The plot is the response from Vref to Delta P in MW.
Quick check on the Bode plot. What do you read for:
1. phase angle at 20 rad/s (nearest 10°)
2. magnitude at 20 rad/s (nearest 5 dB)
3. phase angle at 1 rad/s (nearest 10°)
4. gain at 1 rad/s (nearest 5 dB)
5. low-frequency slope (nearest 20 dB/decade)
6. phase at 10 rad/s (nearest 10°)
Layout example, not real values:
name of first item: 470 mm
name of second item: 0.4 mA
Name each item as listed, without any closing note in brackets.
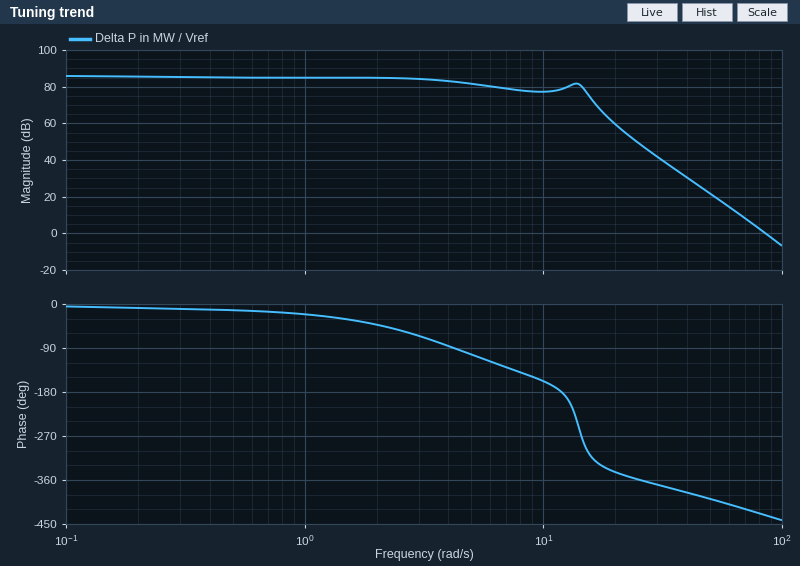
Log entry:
phase angle at 20 rad/s: -340°
magnitude at 20 rad/s: 60 dB
phase angle at 1 rad/s: -20°
gain at 1 rad/s: 85 dB
low-frequency slope: 0 dB/decade
phase at 10 rad/s: -160°
